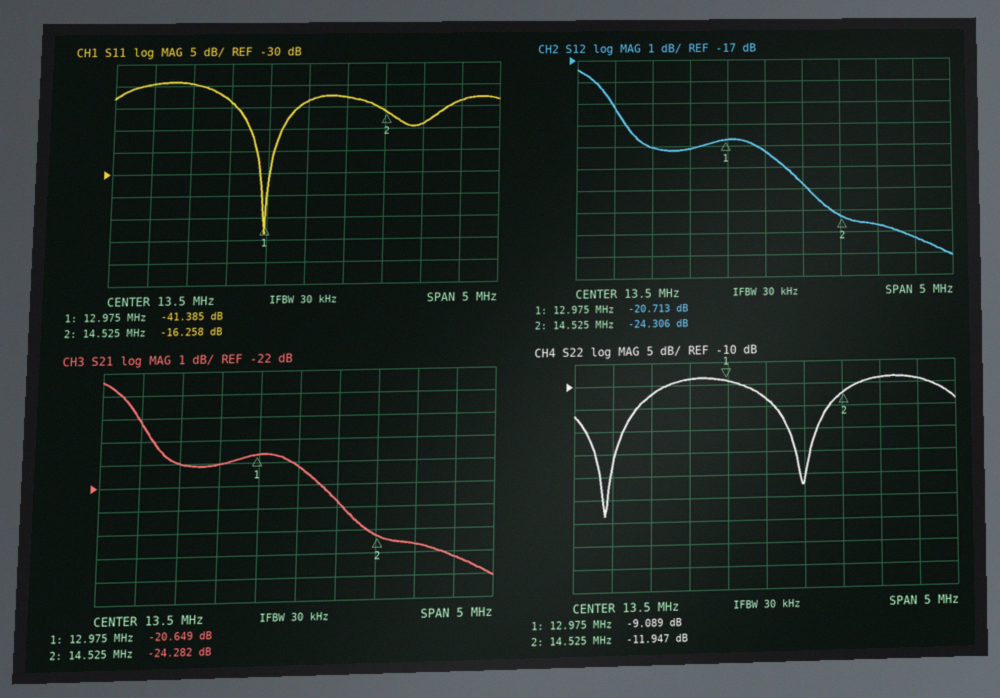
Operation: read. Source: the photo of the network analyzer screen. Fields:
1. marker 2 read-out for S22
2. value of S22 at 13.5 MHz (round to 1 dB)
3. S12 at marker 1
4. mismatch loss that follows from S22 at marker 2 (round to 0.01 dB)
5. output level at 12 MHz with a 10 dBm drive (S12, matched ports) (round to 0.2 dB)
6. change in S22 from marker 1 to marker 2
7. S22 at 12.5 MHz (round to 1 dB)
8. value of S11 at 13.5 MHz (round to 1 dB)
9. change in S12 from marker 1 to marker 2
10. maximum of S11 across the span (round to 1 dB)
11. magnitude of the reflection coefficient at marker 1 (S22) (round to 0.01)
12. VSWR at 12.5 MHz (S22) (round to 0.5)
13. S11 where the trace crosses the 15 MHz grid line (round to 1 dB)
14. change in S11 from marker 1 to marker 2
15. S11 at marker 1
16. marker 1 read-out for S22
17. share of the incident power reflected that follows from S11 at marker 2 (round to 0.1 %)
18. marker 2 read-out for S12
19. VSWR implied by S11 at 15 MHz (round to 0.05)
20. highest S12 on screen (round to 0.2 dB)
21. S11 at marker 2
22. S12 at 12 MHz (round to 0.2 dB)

-11.947 dB
-13 dB
-20.713 dB
0.29 dB
-11.0 dBm
-2.858 dB
-9 dB
-14 dB
-3.593 dB
-9 dB
0.35
2.0
-19 dB
25.127 dB
-41.385 dB
-9.089 dB
2.4 %
-24.306 dB
1.25
-17.4 dB
-16.258 dB
-21.0 dB
